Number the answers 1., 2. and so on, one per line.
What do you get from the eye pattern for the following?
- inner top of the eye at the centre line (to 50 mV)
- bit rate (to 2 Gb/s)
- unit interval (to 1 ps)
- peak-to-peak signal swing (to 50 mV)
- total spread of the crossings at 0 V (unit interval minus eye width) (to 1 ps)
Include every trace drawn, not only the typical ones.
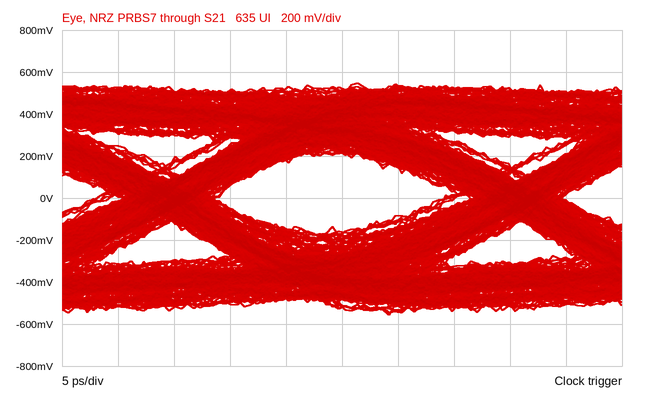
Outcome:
1. 200 mV
2. 32 Gb/s
3. 31 ps
4. 1.10 V
5. 11 ps
